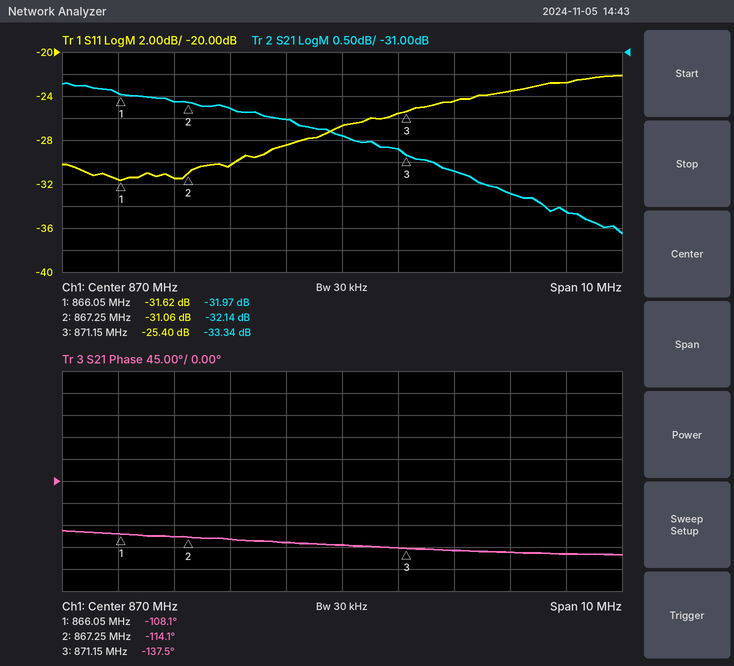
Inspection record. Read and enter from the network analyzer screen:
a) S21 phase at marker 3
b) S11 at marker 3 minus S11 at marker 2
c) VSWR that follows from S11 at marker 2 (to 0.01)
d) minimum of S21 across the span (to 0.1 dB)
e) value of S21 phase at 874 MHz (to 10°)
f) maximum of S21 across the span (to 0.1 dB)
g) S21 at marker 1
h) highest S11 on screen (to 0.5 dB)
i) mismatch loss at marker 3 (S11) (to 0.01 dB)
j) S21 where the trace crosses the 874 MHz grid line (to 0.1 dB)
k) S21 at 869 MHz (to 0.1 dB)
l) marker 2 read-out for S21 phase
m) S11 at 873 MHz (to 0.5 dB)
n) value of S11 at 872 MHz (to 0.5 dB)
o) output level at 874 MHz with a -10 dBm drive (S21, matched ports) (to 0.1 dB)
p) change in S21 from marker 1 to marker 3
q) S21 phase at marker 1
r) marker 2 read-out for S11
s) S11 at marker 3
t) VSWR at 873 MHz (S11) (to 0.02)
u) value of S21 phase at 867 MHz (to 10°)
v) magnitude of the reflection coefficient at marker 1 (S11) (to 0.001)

-137.5°
5.66 dB
1.06
-35.1 dB
-150°
-31.7 dB
-31.97 dB
-22.0 dB
0.01 dB
-34.6 dB
-32.5 dB
-114.1°
-23.5 dB
-24.5 dB
-44.6 dBm
-1.37 dB
-108.1°
-31.06 dB
-25.40 dB
1.14
-110°
0.026
